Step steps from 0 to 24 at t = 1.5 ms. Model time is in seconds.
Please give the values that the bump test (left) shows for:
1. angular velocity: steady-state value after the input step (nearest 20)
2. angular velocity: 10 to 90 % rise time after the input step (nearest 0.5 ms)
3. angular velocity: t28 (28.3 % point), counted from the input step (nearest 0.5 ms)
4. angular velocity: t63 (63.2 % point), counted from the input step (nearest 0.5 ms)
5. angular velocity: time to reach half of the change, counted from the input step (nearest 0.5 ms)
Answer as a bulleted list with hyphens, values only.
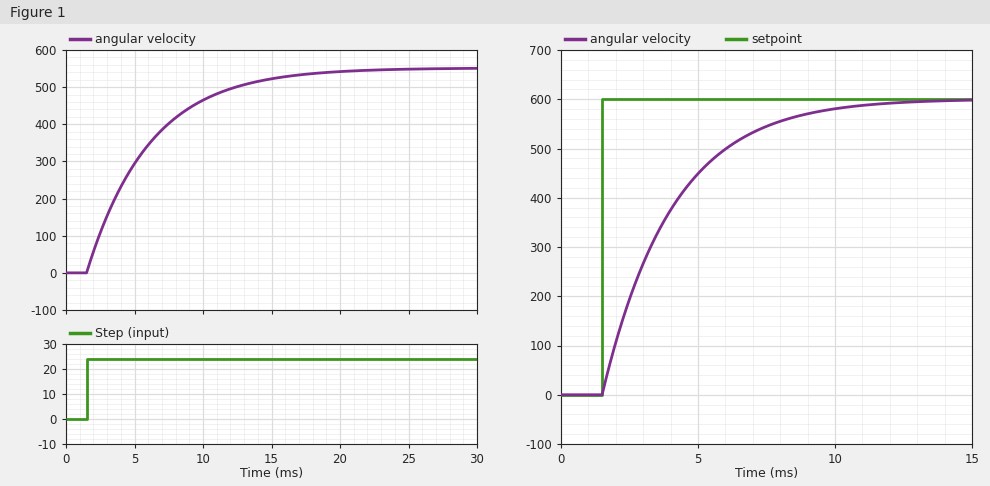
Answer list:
- 560
- 10.0 ms
- 1.5 ms
- 4.5 ms
- 3.0 ms
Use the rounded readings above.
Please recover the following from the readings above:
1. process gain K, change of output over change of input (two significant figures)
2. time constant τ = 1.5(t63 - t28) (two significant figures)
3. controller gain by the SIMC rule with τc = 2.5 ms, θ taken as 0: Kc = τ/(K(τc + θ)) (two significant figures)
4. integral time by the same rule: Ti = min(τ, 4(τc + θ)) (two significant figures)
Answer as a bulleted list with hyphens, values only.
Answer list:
- 23
- 4.5 ms
- 0.078
- 4.5 ms
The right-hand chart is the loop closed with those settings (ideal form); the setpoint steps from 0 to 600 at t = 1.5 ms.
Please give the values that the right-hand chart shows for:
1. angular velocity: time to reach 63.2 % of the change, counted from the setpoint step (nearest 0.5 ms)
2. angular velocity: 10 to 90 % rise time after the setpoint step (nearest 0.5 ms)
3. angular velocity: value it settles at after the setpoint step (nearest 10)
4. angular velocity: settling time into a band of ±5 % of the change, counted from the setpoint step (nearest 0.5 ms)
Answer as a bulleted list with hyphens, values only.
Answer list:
- 2.5 ms
- 5.5 ms
- 600
- 7.5 ms
